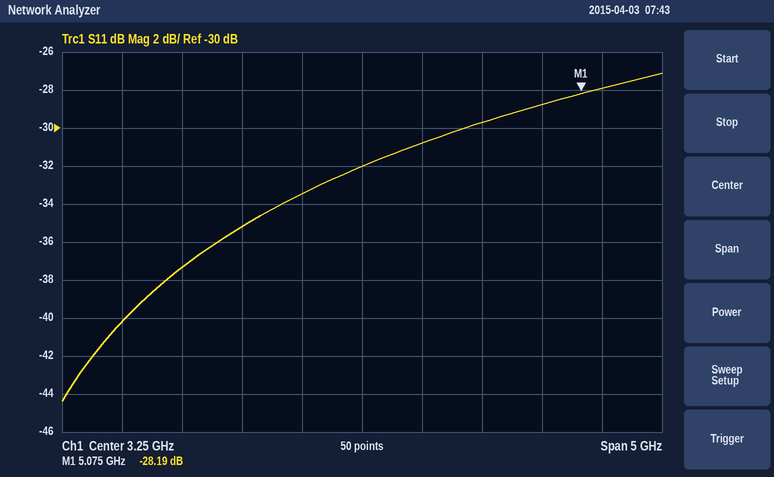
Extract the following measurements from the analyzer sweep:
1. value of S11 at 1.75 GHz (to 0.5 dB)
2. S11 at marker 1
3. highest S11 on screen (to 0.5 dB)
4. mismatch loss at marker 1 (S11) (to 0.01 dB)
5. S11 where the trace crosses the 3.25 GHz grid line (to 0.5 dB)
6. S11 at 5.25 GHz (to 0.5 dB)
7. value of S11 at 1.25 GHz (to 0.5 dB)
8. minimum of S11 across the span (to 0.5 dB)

-37.5 dB
-28.19 dB
-27.0 dB
0.01 dB
-32.0 dB
-28.0 dB
-40.0 dB
-44.5 dB
